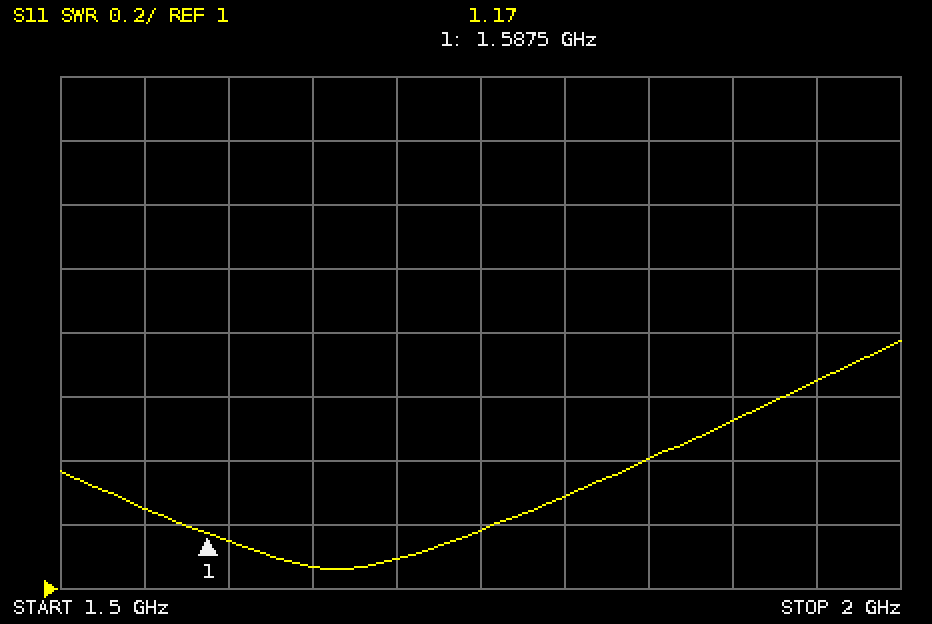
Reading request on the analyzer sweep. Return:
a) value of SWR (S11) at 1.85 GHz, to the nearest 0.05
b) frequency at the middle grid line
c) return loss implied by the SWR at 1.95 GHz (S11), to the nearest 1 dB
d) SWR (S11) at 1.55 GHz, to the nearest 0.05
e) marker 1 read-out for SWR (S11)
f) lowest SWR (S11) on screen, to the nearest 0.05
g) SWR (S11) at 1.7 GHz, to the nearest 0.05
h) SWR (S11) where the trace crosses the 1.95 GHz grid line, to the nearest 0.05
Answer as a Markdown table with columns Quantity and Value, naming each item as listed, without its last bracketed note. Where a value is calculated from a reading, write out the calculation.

| Quantity | Value |
|---|---|
| value of SWR (S11) at 1.85 GHz, to the nearest 0.05 | 1.40 |
| frequency at the middle grid line | 1.75 GHz |
| return loss implied by the SWR at 1.95 GHz (S11), to the nearest 1 dB | −20 log10((1.65 − 1)/(1.65 + 1)) ≈ 12 dB |
| SWR (S11) at 1.55 GHz, to the nearest 0.05 | 1.25 |
| marker 1 read-out for SWR | 1.17 |
| lowest SWR (S11) on screen, to the nearest 0.05 | 1.05 |
| SWR (S11) at 1.7 GHz, to the nearest 0.05 | 1.10 |
| SWR (S11) where the trace crosses the 1.95 GHz grid line, to the nearest 0.05 | 1.65 |
